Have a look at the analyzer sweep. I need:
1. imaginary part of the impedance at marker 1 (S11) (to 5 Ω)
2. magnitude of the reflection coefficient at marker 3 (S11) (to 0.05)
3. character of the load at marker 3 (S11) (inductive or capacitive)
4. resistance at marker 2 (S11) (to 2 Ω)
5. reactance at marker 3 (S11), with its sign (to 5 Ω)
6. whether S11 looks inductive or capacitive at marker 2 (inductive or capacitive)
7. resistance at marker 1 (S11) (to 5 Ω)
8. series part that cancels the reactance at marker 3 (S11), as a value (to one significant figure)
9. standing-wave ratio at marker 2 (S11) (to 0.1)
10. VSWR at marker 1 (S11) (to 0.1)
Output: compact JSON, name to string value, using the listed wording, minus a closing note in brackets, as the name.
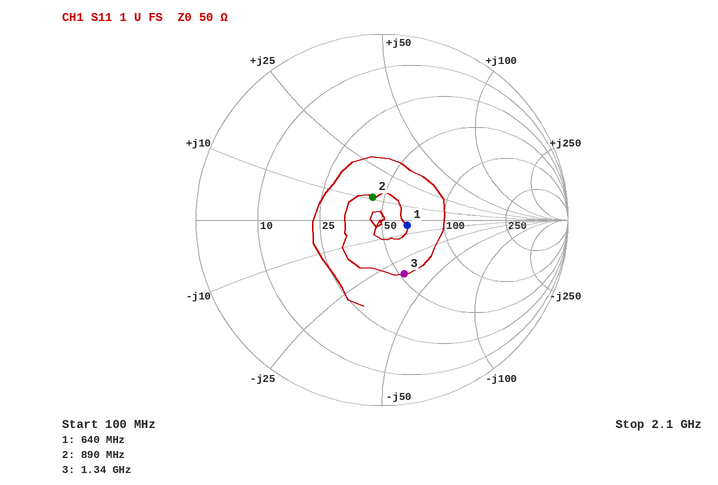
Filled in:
{"imaginary part of the impedance at marker 1 (S11)": "-5 Ω", "magnitude of the reflection coefficient at marker 3 (S11)": "0.30", "character of the load at marker 3 (S11)": "capacitive", "resistance at marker 2 (S11)": "44 Ω", "reactance at marker 3 (S11), with its sign": "-35 Ω", "whether S11 looks inductive or capacitive at marker 2": "inductive", "resistance at marker 1 (S11)": "65 Ω", "series part that cancels the reactance at marker 3 (S11), as a value": "4 nH", "standing-wave ratio at marker 2 (S11)": "1.3", "VSWR at marker 1 (S11)": "1.3"}
